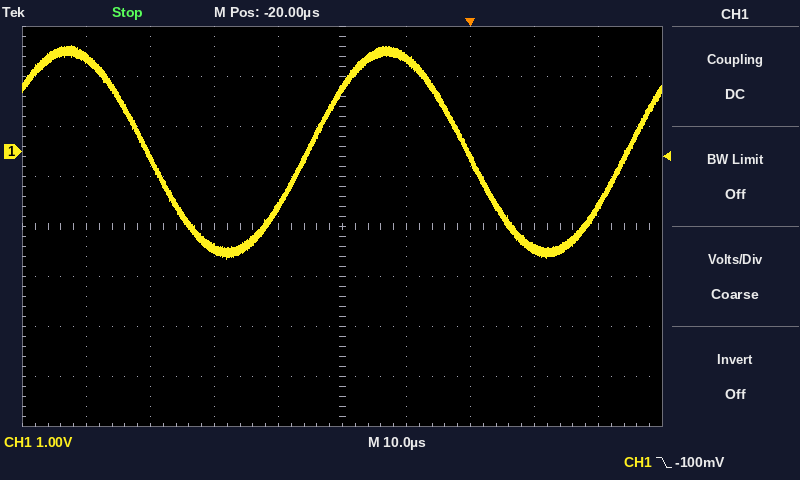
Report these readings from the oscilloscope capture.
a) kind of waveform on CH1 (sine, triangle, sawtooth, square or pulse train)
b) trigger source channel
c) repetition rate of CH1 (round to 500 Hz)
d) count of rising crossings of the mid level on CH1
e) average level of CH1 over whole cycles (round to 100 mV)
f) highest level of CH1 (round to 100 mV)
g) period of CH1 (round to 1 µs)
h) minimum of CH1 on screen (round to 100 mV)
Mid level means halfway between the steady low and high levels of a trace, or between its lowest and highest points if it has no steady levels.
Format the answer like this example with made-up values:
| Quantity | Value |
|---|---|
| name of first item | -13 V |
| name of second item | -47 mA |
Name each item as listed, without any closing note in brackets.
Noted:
| Quantity | Value |
|---|---|
| kind of waveform on CH1 | sine |
| trigger source channel | CH1 |
| repetition rate of CH1 | 20.0 kHz |
| count of rising crossings of the mid level on CH1 | 2 |
| average level of CH1 over whole cycles | 0.0 V |
| highest level of CH1 | 2.1 V |
| period of CH1 | 50 µs |
| minimum of CH1 on screen | -2.1 V |
